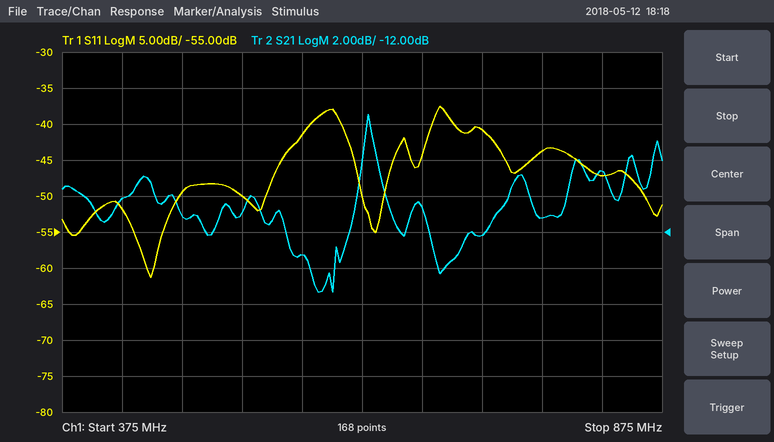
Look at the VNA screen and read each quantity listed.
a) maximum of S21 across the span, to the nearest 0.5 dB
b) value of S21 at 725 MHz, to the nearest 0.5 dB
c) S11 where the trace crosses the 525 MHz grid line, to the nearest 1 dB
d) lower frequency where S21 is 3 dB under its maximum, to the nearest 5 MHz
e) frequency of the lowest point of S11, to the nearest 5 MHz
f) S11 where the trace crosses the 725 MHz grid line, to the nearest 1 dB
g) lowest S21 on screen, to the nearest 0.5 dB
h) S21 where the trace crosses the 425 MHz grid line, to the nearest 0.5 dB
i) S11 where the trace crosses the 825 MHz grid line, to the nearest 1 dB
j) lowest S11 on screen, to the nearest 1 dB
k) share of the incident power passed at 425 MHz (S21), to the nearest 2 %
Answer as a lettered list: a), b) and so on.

a) -5.5 dB
b) -12.0 dB
c) -50 dB
d) 625 MHz
e) 450 MHz
f) -41 dB
g) -15.5 dB
h) -10.0 dB
i) -47 dB
j) -61 dB
k) 10 %
